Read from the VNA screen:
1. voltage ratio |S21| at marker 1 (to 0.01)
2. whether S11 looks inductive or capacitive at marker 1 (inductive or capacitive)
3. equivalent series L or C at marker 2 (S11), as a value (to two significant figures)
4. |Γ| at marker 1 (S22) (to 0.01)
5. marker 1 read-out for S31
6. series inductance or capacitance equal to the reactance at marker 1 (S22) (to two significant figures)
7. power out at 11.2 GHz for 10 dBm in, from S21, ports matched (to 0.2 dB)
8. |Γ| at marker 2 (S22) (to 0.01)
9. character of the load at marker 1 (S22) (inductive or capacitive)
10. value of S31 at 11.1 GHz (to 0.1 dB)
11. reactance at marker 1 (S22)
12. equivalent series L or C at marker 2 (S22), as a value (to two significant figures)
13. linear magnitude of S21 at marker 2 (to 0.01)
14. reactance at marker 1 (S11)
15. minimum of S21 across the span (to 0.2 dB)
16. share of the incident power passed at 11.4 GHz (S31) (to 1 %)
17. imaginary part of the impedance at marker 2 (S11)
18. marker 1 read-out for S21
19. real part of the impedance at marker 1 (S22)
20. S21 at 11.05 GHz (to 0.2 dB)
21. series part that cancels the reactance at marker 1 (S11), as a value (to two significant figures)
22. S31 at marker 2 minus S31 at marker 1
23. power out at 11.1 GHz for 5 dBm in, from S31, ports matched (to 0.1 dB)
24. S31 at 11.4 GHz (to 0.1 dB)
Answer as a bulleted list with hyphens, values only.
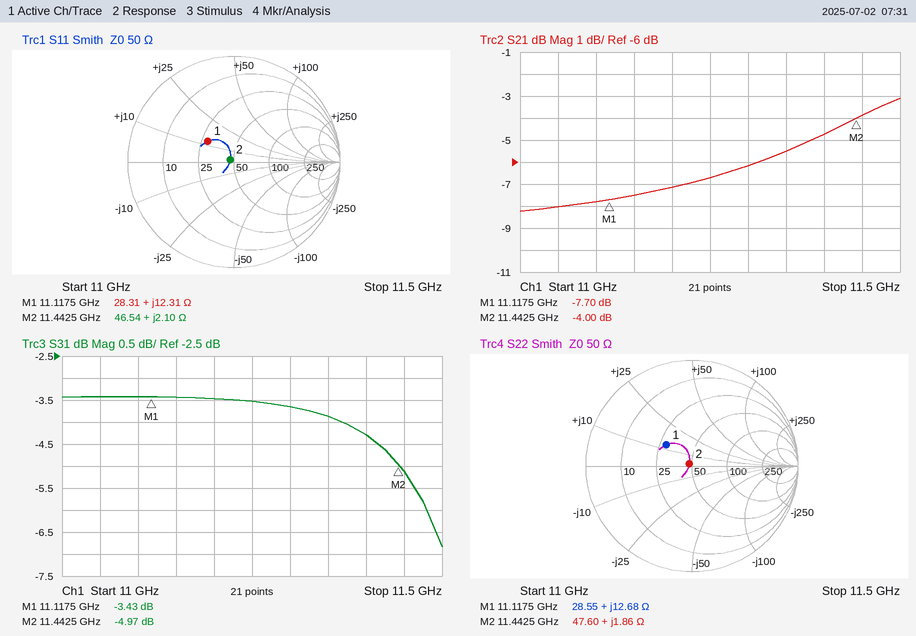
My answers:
- 0.41
- inductive
- 29 pH
- 0.31
- -3.43 dB
- 180 pH
- 2.8 dBm
- 0.03
- inductive
- -3.4 dB
- +12.68 Ω
- 26 pH
- 0.63
- +12.31 Ω
- -8.2 dB
- 37 %
- +2.10 Ω
- -7.70 dB
- 28.55 Ω
- -8.0 dB
- 1.2 pF
- -1.54 dB
- 1.6 dBm
- -4.3 dB
